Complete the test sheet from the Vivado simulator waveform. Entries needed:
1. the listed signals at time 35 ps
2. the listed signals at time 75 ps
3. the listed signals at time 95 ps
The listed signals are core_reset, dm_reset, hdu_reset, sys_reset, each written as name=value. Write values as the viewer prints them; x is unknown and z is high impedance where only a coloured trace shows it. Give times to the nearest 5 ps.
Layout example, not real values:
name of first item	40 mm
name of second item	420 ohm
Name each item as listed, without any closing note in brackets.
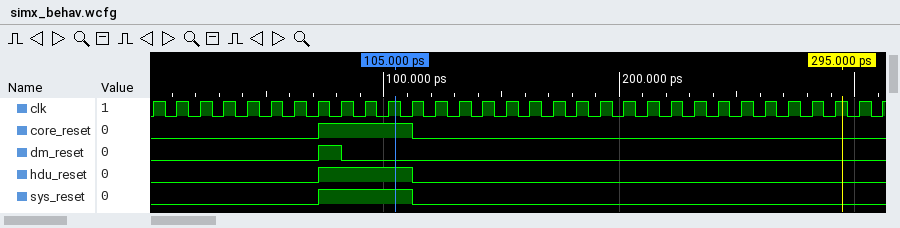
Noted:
the listed signals at time 35 ps	core_reset=0, dm_reset=0, hdu_reset=0, sys_reset=0
the listed signals at time 75 ps	core_reset=1, dm_reset=1, hdu_reset=1, sys_reset=1
the listed signals at time 95 ps	core_reset=1, dm_reset=0, hdu_reset=1, sys_reset=1
